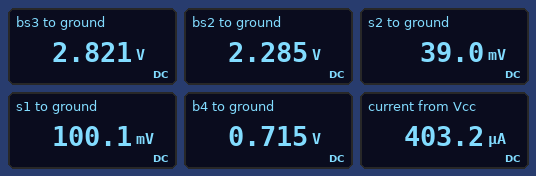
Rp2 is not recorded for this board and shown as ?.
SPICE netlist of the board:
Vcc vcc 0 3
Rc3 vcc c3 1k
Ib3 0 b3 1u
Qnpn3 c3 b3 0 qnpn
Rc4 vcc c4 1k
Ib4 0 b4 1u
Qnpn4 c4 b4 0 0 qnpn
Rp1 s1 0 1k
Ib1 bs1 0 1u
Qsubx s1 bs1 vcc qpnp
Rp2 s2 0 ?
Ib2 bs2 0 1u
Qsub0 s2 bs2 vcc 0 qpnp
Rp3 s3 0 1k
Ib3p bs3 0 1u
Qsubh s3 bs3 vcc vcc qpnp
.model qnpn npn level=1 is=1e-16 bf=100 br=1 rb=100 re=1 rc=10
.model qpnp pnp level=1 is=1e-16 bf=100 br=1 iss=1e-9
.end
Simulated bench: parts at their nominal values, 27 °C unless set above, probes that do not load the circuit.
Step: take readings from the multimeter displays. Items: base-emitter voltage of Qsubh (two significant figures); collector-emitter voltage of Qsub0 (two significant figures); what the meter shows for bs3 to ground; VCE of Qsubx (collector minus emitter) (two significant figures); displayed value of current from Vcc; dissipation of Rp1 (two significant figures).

-180 mV
-3.0 V
2.821 V
-2.9 V
403.2 µA
10 µW
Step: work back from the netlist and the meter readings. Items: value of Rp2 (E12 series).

390 Ω
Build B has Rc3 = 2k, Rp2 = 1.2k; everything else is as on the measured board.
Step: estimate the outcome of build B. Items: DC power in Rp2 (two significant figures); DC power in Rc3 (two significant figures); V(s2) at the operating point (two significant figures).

12 µW
20 µW
120 mV
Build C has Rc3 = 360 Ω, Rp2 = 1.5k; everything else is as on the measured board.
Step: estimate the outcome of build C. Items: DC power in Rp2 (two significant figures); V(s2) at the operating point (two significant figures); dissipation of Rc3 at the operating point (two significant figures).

15 µW
150 mV
3.6 µW
